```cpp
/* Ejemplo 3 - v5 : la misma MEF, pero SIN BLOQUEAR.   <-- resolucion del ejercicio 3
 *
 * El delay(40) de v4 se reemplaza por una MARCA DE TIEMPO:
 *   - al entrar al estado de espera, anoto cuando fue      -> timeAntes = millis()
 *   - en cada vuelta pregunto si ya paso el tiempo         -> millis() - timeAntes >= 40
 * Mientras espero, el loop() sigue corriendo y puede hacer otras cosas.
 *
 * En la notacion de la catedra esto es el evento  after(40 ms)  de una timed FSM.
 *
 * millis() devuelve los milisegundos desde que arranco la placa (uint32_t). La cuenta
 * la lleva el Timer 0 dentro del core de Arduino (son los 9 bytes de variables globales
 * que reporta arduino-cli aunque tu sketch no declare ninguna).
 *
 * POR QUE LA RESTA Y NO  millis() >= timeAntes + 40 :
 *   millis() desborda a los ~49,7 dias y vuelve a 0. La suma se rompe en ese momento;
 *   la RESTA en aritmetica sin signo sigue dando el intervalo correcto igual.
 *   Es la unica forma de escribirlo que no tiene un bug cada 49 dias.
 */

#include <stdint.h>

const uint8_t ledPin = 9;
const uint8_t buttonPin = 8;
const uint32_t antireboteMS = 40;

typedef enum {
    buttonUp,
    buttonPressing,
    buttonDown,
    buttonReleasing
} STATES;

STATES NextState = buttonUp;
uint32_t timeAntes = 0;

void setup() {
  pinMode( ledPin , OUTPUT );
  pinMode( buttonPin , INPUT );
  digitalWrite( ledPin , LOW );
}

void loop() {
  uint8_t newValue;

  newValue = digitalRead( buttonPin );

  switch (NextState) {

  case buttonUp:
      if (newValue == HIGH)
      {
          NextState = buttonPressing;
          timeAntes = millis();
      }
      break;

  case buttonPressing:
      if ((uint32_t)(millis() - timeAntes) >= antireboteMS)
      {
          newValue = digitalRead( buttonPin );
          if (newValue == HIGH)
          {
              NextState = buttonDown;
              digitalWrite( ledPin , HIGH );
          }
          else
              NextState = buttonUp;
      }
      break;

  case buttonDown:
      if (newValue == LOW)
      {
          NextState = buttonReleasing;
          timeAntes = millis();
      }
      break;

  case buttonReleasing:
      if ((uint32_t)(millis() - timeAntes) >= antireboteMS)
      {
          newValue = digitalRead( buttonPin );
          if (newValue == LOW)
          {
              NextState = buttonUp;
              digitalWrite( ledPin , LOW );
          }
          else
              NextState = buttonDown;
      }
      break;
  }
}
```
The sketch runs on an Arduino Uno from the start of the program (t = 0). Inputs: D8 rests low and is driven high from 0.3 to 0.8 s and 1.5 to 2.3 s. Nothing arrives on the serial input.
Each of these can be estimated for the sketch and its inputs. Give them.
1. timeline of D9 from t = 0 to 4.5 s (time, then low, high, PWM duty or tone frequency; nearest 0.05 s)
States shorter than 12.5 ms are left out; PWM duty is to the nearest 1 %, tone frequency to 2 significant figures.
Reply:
0 s low; 0.35 s high; 0.85 s low; 1.55 s high; 2.35 s low
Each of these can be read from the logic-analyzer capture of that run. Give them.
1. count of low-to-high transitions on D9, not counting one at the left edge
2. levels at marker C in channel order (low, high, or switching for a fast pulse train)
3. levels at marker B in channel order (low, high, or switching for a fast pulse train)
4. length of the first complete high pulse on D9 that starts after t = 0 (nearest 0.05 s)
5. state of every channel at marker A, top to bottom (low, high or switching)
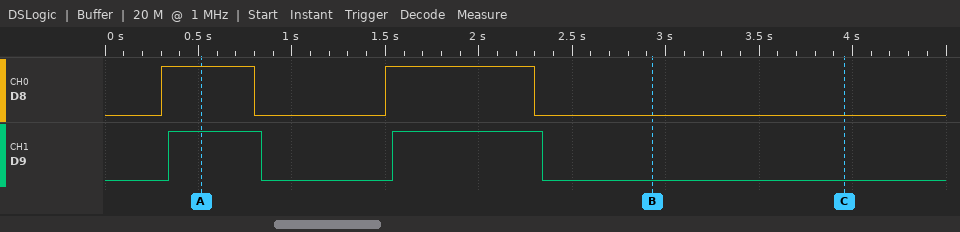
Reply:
2
D8 low, D9 low
D8 low, D9 low
0.50 s
D8 high, D9 high
